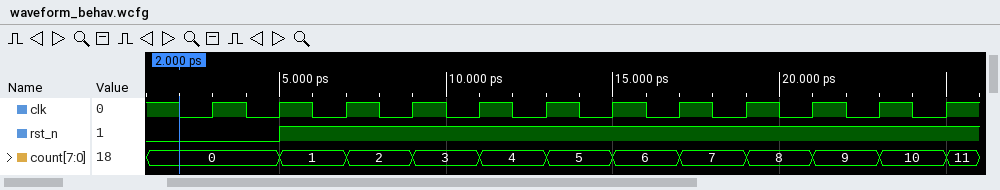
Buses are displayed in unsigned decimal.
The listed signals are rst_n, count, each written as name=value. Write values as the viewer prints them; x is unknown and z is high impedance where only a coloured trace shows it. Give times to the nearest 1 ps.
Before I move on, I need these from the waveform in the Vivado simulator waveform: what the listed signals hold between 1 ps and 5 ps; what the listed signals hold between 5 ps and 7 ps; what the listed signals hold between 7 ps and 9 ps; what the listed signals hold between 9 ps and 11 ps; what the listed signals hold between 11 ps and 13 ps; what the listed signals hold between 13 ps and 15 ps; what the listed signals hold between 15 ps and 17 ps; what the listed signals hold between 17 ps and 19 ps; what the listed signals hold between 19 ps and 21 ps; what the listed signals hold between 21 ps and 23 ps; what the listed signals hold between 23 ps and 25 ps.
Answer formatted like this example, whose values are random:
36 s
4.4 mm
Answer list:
rst_n=0, count=0
rst_n=1, count=1
rst_n=1, count=2
rst_n=1, count=3
rst_n=1, count=4
rst_n=1, count=5
rst_n=1, count=6
rst_n=1, count=7
rst_n=1, count=8
rst_n=1, count=9
rst_n=1, count=10
